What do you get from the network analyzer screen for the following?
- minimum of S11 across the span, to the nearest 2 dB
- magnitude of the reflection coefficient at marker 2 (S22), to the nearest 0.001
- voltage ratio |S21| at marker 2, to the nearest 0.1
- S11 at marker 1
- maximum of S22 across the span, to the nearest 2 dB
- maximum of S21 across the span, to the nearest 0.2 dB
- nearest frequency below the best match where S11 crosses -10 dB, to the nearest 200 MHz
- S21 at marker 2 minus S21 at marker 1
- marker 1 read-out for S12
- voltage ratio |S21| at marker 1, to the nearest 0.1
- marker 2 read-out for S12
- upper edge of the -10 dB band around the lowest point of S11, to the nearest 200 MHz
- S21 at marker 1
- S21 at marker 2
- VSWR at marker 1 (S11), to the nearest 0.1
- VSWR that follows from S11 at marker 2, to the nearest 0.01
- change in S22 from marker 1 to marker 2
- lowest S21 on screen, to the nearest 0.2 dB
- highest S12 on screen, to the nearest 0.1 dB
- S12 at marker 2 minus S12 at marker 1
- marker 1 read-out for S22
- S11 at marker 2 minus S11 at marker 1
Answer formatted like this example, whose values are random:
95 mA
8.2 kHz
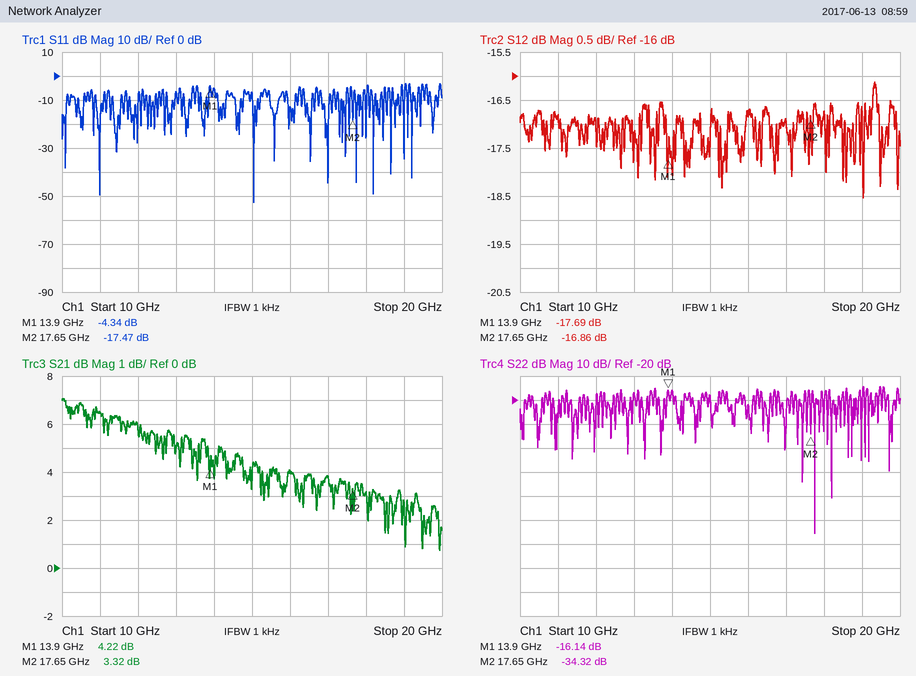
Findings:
-52 dB
0.019
1.5
-4.34 dB
-14 dB
7.0 dB
15.0 GHz
-0.90 dB
-17.69 dB
1.6
-16.86 dB
15.2 GHz
4.22 dB
3.32 dB
4.1
1.31
-18.18 dB
0.8 dB
-16.1 dB
0.83 dB
-16.14 dB
-13.13 dB
